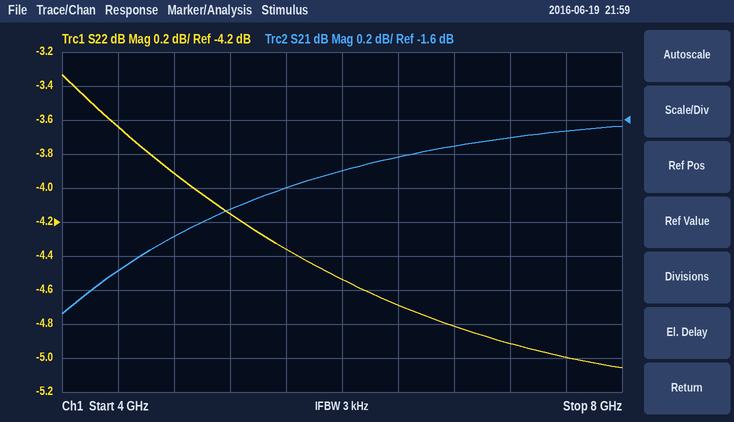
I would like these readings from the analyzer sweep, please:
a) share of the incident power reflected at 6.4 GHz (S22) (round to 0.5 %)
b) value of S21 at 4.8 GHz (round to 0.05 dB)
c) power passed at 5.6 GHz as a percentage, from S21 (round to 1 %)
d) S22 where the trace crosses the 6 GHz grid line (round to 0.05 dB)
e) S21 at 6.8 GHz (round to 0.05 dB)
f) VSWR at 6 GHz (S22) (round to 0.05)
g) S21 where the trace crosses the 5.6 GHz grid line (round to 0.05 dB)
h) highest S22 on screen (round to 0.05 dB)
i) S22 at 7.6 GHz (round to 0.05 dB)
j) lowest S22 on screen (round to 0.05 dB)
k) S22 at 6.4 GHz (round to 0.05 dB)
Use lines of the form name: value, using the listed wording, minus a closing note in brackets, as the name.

share of the incident power reflected at 6.4 GHz (S22): 34.0 %
value of S21 at 4.8 GHz: -2.30 dB
power passed at 5.6 GHz as a percentage, from S21: 63 %
S22 where the trace crosses the 6 GHz grid line: -4.55 dB
S21 at 6.8 GHz: -1.75 dB
VSWR at 6 GHz (S22): 3.90
S21 where the trace crosses the 5.6 GHz grid line: -2.00 dB
highest S22 on screen: -3.35 dB
S22 at 7.6 GHz: -5.00 dB
lowest S22 on screen: -5.05 dB
S22 at 6.4 GHz: -4.70 dB
